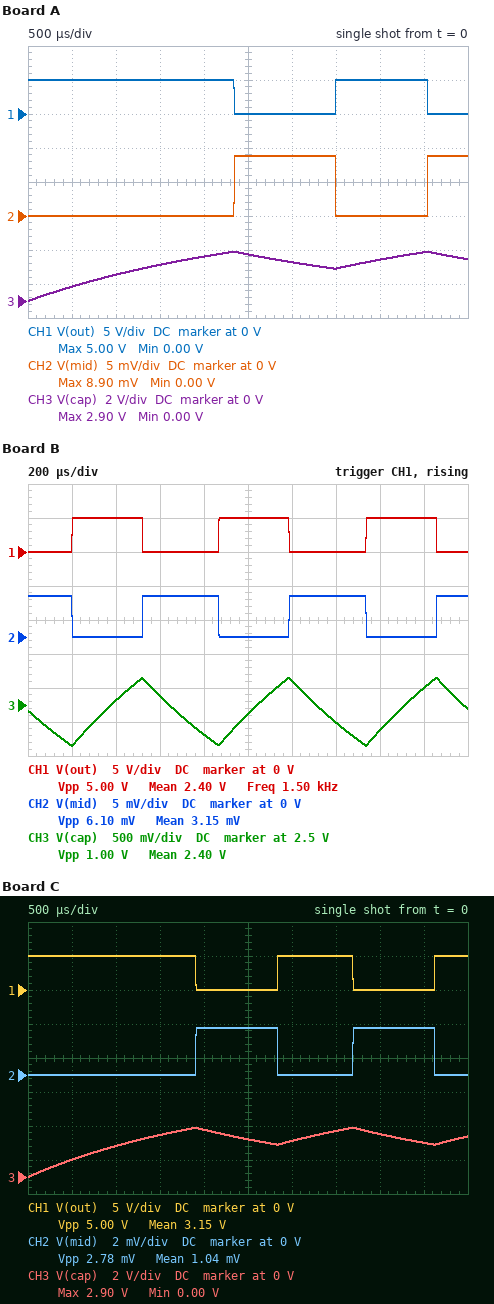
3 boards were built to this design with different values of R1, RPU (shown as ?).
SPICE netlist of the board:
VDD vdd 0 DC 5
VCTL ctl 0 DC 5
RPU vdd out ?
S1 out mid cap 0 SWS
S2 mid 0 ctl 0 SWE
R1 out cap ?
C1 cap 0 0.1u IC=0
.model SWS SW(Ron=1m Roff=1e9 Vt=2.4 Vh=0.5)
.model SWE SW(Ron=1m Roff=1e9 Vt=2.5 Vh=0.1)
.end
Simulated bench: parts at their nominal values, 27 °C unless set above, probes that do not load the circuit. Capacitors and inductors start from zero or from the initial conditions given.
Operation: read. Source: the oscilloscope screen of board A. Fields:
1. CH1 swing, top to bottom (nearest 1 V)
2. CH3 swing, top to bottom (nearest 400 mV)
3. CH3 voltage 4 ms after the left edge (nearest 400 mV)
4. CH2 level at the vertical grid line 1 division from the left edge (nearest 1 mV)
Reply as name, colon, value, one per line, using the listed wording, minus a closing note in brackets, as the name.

CH1 swing, top to bottom: 5 V
CH3 swing, top to bottom: 2.8 V
CH3 voltage 4 ms after the left edge: 2.4 V
CH2 level at the vertical grid line 1 division from the left edge: 0 V
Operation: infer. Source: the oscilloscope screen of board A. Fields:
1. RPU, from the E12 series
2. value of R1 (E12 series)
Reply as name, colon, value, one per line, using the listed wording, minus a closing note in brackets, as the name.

RPU, from the E12 series: 0.56 Ω
value of R1: 27 kΩ
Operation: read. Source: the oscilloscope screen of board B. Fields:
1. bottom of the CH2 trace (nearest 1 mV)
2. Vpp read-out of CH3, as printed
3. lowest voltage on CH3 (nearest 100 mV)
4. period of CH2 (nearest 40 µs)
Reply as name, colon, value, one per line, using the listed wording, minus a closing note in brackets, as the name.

bottom of the CH2 trace: 0 V
Vpp read-out of CH3, as printed: 1.00 V
lowest voltage on CH3: 1.9 V
period of CH2: 680 µs
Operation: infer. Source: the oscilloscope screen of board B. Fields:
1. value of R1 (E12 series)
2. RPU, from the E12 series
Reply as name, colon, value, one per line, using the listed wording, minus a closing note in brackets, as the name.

value of R1: 8.2 kΩ
RPU, from the E12 series: 0.82 Ω
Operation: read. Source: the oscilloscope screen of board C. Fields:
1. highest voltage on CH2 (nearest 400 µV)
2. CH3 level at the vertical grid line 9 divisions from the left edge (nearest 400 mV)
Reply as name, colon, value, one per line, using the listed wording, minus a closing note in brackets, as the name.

highest voltage on CH2: 2.8 mV
CH3 level at the vertical grid line 9 divisions from the left edge: 2.0 V
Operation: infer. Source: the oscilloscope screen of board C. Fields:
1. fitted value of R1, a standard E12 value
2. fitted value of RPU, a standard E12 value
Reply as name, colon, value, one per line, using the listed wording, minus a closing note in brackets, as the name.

fitted value of R1, a standard E12 value: 22 kΩ
fitted value of RPU, a standard E12 value: 1.8 Ω
